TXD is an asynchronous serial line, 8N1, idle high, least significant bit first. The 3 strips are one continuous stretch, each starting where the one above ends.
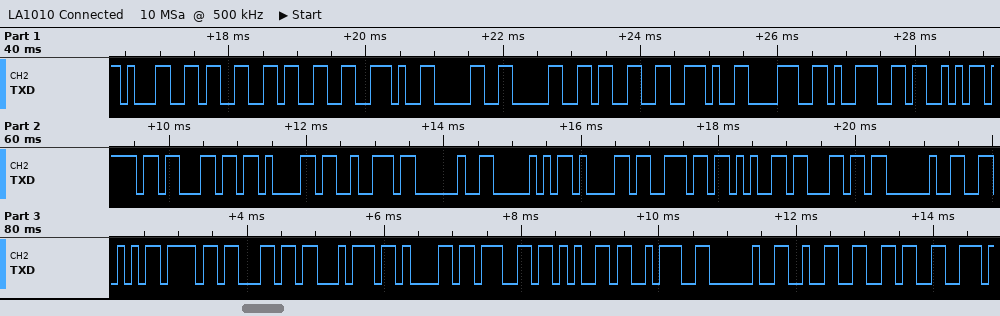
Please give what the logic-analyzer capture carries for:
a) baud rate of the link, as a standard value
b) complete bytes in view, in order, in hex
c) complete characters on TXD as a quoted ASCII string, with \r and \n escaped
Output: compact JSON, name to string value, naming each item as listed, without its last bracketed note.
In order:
{"baud rate of the link, as a standard value": "9600 baud", "complete bytes in view, in order, in hex": "31 33 33 2E 30 30 33 2E 38 39 53 6F 6C 61 72 20 50 61 6E 65 6C 20 56 6F 6C 74 61 67 65 3A 20 32 36", "complete characters on TXD as a quoted ASCII string, with \\r and \\n escaped": "\"133.003.89Solar Panel Voltage: 26\""}
